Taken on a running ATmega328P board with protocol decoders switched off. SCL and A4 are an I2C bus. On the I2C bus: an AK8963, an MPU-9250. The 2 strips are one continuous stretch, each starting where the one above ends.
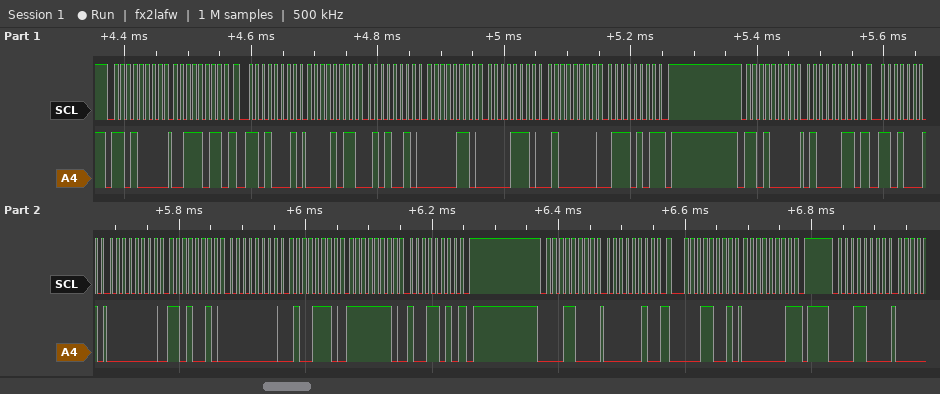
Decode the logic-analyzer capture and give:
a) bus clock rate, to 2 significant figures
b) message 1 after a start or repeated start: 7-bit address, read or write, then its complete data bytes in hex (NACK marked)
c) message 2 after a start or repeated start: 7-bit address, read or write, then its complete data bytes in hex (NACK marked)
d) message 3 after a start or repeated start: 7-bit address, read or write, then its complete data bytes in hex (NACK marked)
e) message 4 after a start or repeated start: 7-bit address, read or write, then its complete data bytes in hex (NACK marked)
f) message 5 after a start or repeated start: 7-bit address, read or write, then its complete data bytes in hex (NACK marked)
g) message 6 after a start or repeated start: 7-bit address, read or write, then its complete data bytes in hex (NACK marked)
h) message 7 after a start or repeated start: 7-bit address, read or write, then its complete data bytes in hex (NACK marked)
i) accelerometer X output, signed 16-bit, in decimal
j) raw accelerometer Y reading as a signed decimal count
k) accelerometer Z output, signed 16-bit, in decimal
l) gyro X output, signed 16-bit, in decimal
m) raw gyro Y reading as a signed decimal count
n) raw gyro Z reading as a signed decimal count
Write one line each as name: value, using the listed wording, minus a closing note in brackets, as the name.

bus clock rate, to 2 significant figures: 100 kHz
message 1 after a start or repeated start: 7-bit address, read or write, then its complete data bytes in hex: 0x68 write: 3B
message 2 after a start or repeated start: 7-bit address, read or write, then its complete data bytes in hex: 0x68 read: 0B 52 06 0E 40 75 NACK
message 3 after a start or repeated start: 7-bit address, read or write, then its complete data bytes in hex: 0x68 write: 43
message 4 after a start or repeated start: 7-bit address, read or write, then its complete data bytes in hex: 0x68 read: 00 D2 00 4E FE 9A NACK
message 5 after a start or repeated start: 7-bit address, read or write, then its complete data bytes in hex: 0x0C write: 02
message 6 after a start or repeated start: 7-bit address, read or write, then its complete data bytes in hex: 0x0C read: 01 NACK
message 7 after a start or repeated start: 7-bit address, read or write, then its complete data bytes in hex: 0x0C write
accelerometer X output, signed 16-bit, in decimal: 2898
raw accelerometer Y reading as a signed decimal count: 1550
accelerometer Z output, signed 16-bit, in decimal: 16501
gyro X output, signed 16-bit, in decimal: 210
raw gyro Y reading as a signed decimal count: 78
raw gyro Z reading as a signed decimal count: -358
